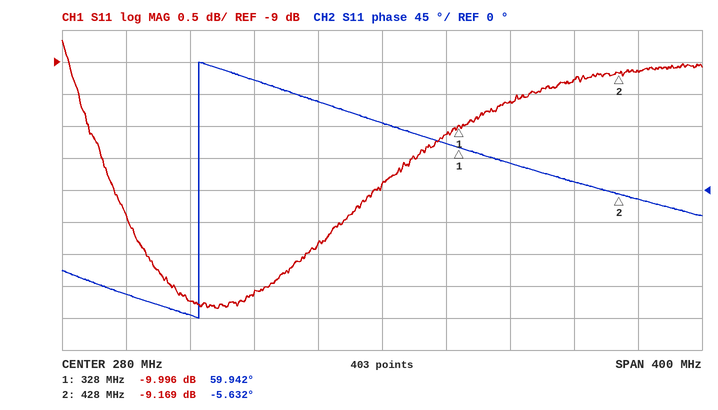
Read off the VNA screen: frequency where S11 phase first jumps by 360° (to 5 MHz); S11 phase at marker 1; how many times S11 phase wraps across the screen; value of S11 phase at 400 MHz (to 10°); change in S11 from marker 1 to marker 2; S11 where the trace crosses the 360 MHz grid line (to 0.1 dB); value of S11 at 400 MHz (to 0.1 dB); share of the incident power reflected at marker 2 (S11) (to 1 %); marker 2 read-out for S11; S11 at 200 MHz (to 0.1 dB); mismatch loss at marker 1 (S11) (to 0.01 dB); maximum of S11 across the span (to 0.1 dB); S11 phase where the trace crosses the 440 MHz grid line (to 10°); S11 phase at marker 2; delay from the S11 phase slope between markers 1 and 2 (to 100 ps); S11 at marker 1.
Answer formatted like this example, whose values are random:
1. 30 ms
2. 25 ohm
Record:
1. 165 MHz
2. 59.942°
3. 1
4. 10°
5. 0.827 dB
6. -9.6 dB
7. -9.3 dB
8. 12 %
9. -9.169 dB
10. -12.6 dB
11. 0.46 dB
12. -8.7 dB
13. -10°
14. -5.632°
15. 1.8 ns
16. -9.996 dB
